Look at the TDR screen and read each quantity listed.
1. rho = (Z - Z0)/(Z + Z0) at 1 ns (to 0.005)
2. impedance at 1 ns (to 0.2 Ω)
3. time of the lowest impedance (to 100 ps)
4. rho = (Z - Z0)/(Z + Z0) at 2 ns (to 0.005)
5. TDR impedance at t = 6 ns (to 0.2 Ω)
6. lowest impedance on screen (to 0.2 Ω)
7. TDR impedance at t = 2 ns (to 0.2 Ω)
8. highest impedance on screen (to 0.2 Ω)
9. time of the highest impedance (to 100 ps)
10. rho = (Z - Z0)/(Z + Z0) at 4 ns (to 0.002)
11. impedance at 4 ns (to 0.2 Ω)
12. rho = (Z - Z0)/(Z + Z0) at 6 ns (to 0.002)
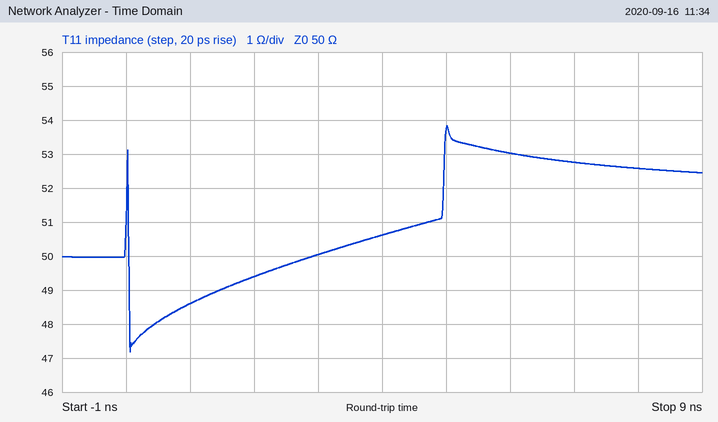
-0.015
48.6 Ω
100 ps
-0.005
53.0 Ω
47.2 Ω
49.4 Ω
53.8 Ω
5.0 ns
+0.006
50.6 Ω
+0.030
